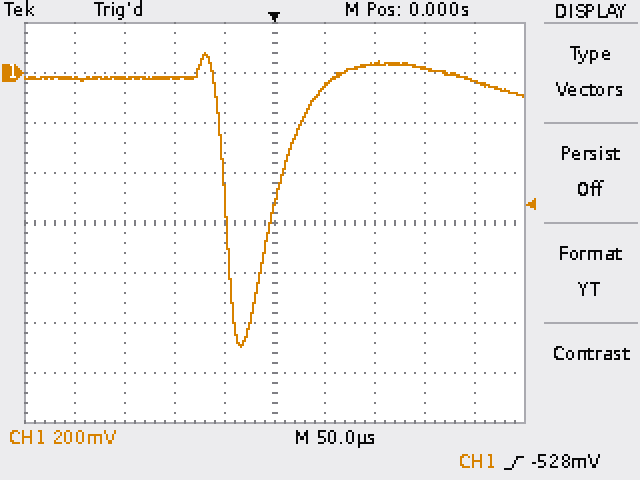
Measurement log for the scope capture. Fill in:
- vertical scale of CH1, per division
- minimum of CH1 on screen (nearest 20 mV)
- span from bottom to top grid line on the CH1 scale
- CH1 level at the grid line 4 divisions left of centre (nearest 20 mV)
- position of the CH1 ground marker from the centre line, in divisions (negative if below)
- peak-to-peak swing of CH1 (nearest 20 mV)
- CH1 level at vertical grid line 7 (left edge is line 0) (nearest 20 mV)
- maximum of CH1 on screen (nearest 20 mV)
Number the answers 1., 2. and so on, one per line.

1. 200 mV
2. -1.10 V
3. 1.6 V
4. -20 mV
5. +3.0 div
6. 1.18 V
7. 40 mV
8. 80 mV
